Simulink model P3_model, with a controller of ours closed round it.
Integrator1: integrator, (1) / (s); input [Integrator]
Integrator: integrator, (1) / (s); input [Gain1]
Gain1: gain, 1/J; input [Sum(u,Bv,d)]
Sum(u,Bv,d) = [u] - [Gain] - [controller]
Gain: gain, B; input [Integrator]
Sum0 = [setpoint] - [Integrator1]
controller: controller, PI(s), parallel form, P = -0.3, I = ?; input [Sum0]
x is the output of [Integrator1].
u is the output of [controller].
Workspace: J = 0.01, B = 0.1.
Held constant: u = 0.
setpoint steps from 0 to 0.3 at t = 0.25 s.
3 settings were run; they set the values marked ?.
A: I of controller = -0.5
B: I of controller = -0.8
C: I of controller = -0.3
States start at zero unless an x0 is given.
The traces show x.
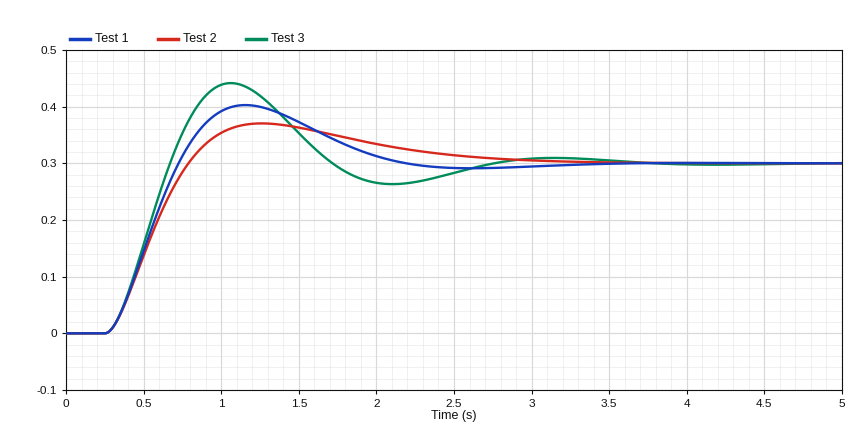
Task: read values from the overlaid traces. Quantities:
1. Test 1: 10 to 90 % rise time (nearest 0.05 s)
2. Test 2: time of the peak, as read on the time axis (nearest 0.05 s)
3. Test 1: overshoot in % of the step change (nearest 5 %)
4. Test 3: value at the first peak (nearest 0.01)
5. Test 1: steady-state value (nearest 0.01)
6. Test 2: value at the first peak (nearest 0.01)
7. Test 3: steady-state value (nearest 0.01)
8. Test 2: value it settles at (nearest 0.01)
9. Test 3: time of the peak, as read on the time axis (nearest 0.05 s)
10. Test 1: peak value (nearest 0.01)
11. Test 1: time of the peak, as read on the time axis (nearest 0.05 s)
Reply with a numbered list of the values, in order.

1. 0.35 s
2. 1.25 s
3. 35 %
4. 0.44
5. 0.30
6. 0.37
7. 0.30
8. 0.30
9. 1.05 s
10. 0.40
11. 1.15 s
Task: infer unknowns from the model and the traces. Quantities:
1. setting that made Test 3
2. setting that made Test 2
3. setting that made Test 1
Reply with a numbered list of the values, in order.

1. B
2. C
3. A
